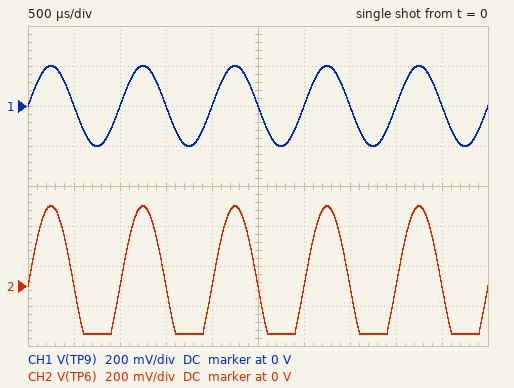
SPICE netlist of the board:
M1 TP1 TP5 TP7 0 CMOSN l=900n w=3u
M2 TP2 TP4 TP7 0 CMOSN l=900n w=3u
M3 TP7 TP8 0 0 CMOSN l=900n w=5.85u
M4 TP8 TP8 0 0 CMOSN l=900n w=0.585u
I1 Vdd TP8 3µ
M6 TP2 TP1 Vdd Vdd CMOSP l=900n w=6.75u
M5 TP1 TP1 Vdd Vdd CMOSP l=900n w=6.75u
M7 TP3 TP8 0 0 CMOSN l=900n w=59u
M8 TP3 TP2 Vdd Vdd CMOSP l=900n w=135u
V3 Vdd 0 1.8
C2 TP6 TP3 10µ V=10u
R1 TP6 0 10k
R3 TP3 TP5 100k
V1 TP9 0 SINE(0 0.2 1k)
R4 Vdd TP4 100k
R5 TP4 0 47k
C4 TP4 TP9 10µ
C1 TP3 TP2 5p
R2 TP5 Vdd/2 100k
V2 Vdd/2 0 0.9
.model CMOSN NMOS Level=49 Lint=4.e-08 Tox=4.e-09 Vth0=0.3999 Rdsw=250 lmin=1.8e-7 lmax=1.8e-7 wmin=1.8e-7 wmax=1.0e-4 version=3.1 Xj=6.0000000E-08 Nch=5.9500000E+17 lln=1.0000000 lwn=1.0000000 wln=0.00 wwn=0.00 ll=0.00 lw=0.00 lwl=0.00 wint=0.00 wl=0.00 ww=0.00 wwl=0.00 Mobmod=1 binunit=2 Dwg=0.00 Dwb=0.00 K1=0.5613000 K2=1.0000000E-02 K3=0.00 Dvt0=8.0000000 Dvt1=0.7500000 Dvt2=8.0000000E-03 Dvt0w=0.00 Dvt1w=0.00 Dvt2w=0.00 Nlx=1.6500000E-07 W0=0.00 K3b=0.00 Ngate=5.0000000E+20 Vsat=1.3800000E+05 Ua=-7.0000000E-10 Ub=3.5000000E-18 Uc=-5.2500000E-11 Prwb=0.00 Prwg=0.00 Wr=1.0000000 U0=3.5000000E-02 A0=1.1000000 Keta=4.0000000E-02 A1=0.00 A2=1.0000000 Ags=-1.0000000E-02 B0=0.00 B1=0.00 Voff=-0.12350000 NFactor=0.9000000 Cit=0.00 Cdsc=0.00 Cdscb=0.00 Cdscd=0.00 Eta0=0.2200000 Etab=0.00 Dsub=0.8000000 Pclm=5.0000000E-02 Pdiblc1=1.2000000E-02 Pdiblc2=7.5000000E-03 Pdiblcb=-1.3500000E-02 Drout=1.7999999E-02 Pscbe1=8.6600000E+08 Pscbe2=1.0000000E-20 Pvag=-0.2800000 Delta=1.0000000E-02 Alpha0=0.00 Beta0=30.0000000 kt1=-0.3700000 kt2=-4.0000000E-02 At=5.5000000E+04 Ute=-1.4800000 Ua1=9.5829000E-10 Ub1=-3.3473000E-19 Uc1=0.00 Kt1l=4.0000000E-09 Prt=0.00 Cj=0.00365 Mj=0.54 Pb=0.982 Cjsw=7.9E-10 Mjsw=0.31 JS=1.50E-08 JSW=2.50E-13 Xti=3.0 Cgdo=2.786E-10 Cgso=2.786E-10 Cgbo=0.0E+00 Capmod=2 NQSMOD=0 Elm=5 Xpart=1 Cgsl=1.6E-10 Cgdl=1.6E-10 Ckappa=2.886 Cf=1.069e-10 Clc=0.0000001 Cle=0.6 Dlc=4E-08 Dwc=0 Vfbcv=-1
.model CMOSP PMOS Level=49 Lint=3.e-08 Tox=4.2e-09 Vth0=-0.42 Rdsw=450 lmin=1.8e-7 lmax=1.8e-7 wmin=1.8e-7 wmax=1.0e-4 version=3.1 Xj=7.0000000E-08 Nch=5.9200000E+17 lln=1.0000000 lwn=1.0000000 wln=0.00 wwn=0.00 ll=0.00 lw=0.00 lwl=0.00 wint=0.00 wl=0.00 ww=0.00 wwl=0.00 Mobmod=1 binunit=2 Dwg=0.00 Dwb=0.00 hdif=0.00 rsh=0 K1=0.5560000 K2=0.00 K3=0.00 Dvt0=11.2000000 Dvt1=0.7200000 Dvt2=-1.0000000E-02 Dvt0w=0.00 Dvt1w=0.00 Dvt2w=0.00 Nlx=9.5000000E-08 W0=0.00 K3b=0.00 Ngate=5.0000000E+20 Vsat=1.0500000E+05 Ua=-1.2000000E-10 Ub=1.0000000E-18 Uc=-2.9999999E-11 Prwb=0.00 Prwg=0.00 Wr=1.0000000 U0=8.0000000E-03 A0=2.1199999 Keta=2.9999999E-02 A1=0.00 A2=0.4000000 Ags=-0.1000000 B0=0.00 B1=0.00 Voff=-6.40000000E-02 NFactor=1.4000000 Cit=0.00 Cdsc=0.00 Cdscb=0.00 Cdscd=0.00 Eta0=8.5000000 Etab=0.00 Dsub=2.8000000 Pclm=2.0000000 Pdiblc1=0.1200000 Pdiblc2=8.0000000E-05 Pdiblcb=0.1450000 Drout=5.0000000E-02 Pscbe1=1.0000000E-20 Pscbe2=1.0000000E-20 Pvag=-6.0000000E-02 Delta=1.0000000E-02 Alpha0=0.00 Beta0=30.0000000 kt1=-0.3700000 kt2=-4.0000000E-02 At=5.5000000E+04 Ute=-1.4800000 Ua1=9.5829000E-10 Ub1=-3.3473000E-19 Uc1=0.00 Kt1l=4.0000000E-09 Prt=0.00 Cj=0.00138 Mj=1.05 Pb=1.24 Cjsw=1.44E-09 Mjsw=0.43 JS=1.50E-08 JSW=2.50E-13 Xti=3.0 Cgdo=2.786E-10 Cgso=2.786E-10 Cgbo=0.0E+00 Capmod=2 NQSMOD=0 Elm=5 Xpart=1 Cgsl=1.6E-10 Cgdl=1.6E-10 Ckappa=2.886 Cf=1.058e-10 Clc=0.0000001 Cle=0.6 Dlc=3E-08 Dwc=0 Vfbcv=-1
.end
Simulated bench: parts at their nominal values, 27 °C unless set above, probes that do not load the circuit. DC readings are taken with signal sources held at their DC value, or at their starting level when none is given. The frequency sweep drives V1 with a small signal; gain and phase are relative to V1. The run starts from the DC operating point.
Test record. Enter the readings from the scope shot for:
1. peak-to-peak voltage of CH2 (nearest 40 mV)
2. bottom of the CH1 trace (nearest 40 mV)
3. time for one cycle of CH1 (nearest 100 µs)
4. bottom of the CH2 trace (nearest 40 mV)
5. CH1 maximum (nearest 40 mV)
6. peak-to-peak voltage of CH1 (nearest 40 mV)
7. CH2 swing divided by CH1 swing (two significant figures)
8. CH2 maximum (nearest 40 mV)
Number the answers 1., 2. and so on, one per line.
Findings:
1. 640 mV
2. -200 mV
3. 1.0 ms
4. -240 mV
5. 200 mV
6. 400 mV
7. 1.6
8. 400 mV
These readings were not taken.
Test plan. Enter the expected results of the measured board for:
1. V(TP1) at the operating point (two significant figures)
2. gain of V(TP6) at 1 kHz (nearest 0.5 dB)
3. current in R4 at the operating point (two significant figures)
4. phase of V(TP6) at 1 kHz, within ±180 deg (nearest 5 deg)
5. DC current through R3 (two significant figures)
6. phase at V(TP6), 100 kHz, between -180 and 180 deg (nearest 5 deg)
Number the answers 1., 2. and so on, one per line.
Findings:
1. 1.2 V
2. 6.0 dB
3. 12 µA
4. 0 deg
5. 3.3 µA
6. -5 deg
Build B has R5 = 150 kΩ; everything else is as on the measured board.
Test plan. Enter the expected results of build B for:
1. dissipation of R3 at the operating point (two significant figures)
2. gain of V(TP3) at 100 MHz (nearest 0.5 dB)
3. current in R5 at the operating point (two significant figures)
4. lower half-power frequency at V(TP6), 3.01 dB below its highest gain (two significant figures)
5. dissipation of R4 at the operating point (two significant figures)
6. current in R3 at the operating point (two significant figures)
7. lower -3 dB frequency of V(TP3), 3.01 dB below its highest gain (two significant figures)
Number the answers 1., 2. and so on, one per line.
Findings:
1. 320 nW
2. -25.5 dB
3. 7.2 µA
4. 1.6 Hz
5. 5.2 µW
6. 1.8 µA
7. 260 mHz
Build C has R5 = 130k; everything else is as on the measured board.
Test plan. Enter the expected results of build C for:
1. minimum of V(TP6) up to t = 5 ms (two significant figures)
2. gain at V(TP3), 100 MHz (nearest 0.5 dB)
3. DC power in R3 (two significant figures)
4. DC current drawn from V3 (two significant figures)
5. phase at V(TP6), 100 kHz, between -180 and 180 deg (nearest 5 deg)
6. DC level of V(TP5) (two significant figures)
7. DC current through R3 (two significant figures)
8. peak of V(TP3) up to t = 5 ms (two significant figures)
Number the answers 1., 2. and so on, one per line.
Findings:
1. -400 mV
2. -25.5 dB
3. 140 nW
4. 360 µA
5. -5 deg
6. 1.0 V
7. 1.2 µA
8. 1.5 V
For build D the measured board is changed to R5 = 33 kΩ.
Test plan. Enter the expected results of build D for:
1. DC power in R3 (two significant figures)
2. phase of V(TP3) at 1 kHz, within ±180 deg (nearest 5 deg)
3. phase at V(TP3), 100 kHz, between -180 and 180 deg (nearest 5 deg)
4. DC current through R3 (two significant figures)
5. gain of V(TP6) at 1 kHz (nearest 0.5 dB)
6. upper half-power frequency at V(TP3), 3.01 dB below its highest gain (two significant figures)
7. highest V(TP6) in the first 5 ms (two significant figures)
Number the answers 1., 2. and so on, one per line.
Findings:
1. 2.0 µW
2. -5 deg
3. -150 deg
4. 4.5 µA
5. -31.5 dB
6. 13 kHz
7. 390 mV
